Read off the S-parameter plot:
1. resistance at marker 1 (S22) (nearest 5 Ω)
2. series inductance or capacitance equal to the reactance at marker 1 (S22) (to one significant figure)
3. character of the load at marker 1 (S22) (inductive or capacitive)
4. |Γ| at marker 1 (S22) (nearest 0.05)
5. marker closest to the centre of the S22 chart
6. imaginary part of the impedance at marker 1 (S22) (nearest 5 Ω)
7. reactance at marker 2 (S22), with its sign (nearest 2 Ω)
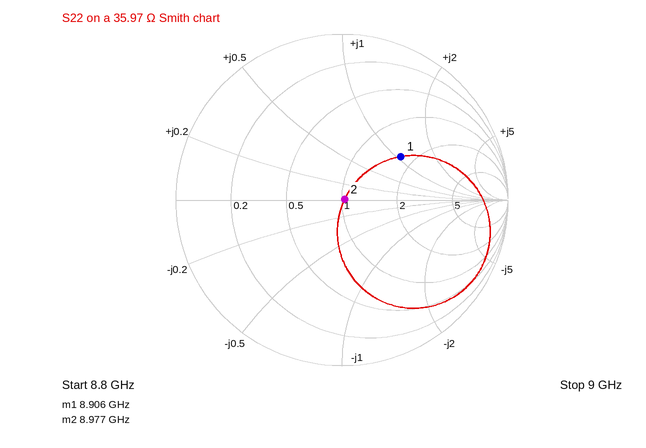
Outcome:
60 Ω
700 pH
inductive
0.45
marker 2
+40 Ω
0 Ω
